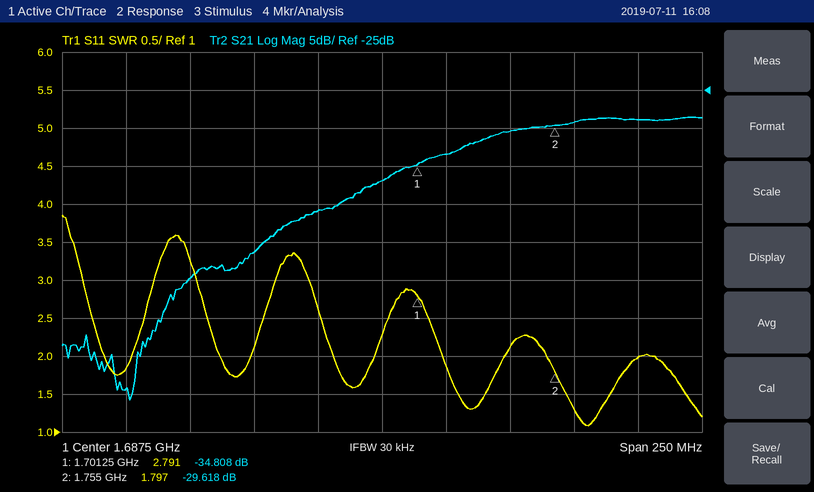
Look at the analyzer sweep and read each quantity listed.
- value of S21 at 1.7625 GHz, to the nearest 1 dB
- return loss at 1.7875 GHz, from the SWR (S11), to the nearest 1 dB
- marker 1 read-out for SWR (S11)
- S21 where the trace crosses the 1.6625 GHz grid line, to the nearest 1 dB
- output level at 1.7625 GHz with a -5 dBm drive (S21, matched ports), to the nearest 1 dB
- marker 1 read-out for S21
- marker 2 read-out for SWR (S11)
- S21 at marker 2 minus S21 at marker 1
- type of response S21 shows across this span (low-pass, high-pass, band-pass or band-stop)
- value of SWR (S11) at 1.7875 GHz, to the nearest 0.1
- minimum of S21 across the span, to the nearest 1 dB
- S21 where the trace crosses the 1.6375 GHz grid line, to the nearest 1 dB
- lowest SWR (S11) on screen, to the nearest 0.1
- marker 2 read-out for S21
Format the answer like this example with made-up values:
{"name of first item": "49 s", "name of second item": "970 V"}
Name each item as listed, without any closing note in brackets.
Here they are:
{"value of S21 at 1.7625 GHz, to the nearest 1 dB": "-29 dB", "return loss at 1.7875 GHz, from the SWR (S11), to the nearest 1 dB": "10 dB", "marker 1 read-out for SWR": "2.791", "S21 where the trace crosses the 1.6625 GHz grid line, to the nearest 1 dB": "-41 dB", "output level at 1.7625 GHz with a -5 dBm drive (S21, matched ports), to the nearest 1 dB": "-34 dBm", "marker 1 read-out for S21": "-34.808 dB", "marker 2 read-out for SWR": "1.797", "S21 at marker 2 minus S21 at marker 1": "5.190 dB", "type of response S21 shows across this span": "high-pass", "value of SWR (S11) at 1.7875 GHz, to the nearest 0.1": "2.0", "minimum of S21 across the span, to the nearest 1 dB": "-66 dB", "S21 where the trace crosses the 1.6375 GHz grid line, to the nearest 1 dB": "-46 dB", "lowest SWR (S11) on screen, to the nearest 0.1": "1.1", "marker 2 read-out for S21": "-29.618 dB"}
